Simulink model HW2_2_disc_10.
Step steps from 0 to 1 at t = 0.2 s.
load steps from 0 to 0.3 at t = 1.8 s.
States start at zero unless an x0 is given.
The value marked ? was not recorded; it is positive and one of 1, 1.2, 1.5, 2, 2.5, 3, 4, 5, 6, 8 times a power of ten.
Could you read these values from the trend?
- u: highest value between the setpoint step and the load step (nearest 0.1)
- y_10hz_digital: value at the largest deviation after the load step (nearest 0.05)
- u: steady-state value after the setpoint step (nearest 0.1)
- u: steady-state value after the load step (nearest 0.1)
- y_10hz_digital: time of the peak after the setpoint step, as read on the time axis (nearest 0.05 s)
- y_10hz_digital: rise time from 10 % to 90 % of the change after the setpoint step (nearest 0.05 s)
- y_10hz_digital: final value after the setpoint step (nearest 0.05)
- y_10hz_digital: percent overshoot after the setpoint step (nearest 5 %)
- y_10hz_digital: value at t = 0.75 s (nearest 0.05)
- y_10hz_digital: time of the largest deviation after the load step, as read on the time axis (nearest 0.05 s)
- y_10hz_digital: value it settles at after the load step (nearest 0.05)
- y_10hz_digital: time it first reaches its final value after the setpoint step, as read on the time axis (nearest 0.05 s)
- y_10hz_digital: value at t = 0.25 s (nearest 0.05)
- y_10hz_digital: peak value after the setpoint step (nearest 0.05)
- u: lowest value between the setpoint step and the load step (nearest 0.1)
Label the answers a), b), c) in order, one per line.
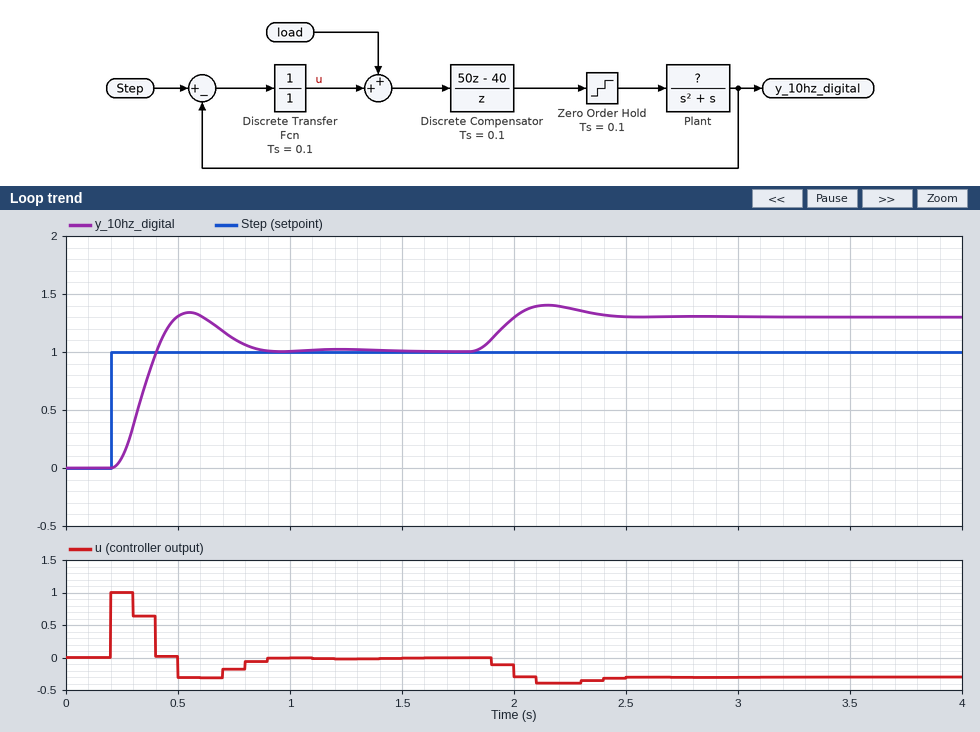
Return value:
a) 1.0
b) 1.40
c) 0.0
d) -0.3
e) 0.55 s
f) 0.15 s
g) 1.00
h) 35 %
i) 1.10
j) 2.15 s
k) 1.30
l) 0.40 s
m) 0.10
n) 1.35
o) -0.3
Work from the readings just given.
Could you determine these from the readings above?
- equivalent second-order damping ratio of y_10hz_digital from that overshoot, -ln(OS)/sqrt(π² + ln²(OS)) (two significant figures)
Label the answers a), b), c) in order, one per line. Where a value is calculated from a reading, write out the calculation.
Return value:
a) ln(0.35) = -1.050; 1.050 / sqrt(9.870 + 1.102) = 0.32
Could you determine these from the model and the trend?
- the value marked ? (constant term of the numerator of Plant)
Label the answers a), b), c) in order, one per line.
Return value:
a) 1.5
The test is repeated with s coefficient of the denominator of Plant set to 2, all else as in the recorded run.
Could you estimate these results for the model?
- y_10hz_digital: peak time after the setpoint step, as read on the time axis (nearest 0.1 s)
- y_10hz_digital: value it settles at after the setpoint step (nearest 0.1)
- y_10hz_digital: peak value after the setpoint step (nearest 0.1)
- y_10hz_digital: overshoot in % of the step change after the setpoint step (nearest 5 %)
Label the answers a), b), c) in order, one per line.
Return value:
a) 0.5 s
b) 1.0
c) 1.2
d) 20 %
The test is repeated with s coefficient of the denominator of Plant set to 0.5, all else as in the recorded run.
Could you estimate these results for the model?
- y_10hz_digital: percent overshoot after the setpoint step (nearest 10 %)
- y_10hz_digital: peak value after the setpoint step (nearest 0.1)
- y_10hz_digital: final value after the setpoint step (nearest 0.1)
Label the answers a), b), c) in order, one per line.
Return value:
a) 40 %
b) 1.4
c) 1.0
